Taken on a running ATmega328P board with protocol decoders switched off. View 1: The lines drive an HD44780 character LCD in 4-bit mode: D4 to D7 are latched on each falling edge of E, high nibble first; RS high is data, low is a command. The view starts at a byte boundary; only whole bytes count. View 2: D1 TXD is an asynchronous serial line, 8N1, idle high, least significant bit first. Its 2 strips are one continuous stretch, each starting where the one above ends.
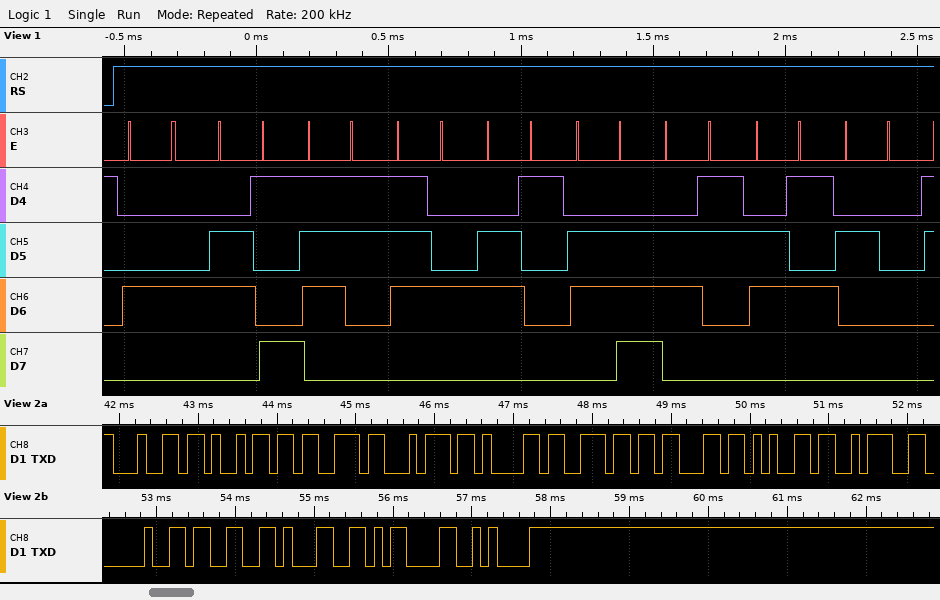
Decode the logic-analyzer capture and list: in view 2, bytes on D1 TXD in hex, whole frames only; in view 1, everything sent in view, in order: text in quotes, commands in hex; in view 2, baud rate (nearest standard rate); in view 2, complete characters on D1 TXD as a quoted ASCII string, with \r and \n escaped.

0x64 0x69 0x73 0x74 0x61 0x6E 0x63 0x65 0x3A 0x20 0x33 0x31 0x0D 0x0A
"Distance "
9600 baud
"distance: 31\r\n"
